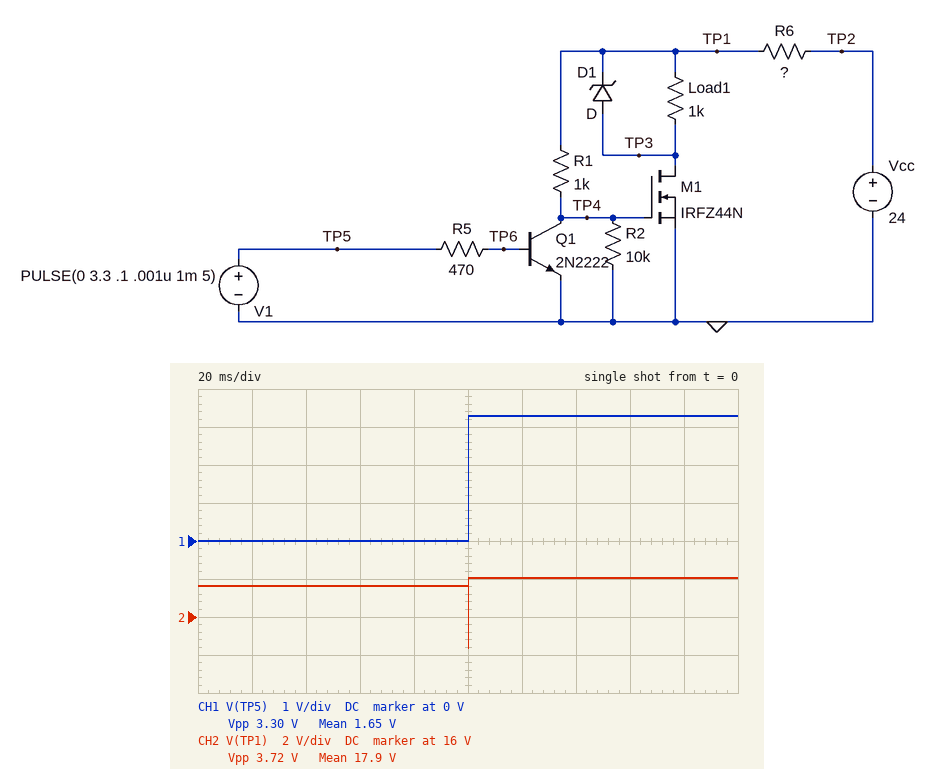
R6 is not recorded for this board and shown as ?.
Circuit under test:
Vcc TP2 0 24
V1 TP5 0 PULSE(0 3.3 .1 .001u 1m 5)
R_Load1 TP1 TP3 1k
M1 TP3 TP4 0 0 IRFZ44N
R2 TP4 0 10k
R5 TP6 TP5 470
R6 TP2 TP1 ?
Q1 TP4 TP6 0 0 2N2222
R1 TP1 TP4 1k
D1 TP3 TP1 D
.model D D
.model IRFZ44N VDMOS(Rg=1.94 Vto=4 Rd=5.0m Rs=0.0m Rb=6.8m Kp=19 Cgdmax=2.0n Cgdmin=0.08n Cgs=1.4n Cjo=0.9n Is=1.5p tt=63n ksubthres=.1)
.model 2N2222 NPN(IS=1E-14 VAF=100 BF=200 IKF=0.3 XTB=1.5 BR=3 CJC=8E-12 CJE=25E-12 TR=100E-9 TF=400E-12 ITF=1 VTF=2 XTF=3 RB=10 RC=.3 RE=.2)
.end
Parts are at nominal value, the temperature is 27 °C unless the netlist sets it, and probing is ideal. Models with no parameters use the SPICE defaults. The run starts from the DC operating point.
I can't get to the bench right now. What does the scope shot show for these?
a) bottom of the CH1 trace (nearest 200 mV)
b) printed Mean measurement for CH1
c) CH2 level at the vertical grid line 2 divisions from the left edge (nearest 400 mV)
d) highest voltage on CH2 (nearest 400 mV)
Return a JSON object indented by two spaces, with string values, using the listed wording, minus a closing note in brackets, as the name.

{
  "bottom of the CH1 trace": "0 V",
  "printed Mean measurement for CH1": "1.65 V",
  "CH2 level at the vertical grid line 2 divisions from the left edge": "17.6 V",
  "highest voltage on CH2": "18.0 V"
}
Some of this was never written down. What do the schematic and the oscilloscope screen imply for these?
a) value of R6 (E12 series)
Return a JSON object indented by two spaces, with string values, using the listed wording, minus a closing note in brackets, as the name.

{
  "value of R6": "330 Ω"
}
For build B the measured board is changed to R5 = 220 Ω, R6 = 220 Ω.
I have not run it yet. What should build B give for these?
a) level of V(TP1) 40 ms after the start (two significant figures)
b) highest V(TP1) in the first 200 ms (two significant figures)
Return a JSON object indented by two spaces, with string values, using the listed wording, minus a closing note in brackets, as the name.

{
  "level of V(TP1) 40 ms after the start": "19 V",
  "highest V(TP1) in the first 200 ms": "20 V"
}
